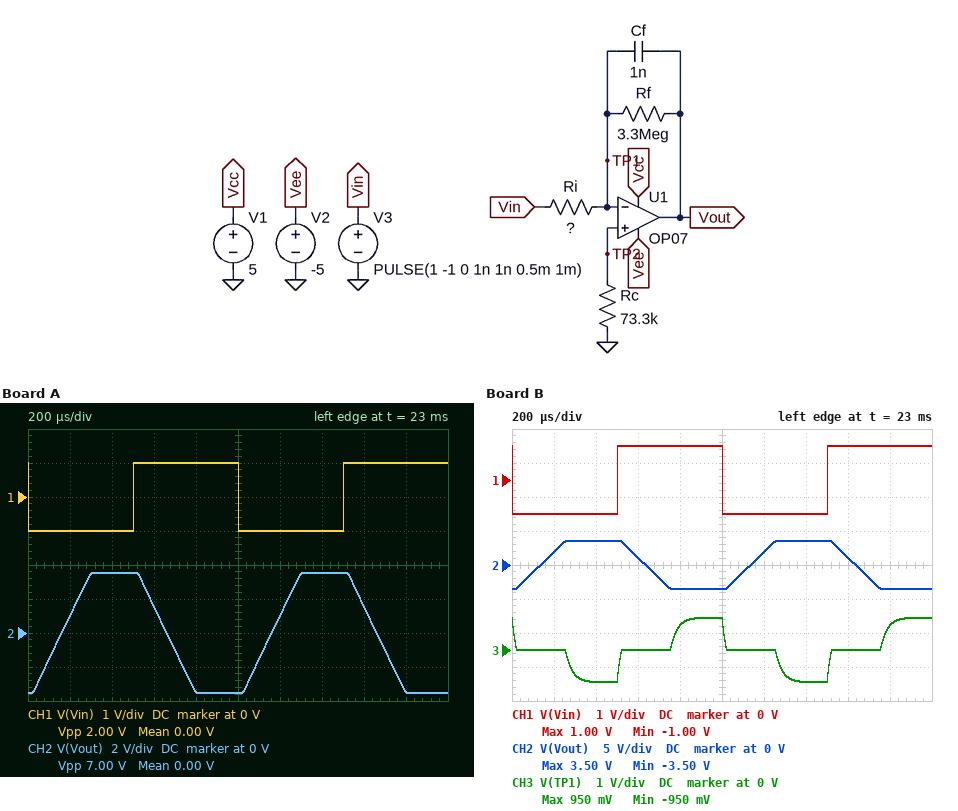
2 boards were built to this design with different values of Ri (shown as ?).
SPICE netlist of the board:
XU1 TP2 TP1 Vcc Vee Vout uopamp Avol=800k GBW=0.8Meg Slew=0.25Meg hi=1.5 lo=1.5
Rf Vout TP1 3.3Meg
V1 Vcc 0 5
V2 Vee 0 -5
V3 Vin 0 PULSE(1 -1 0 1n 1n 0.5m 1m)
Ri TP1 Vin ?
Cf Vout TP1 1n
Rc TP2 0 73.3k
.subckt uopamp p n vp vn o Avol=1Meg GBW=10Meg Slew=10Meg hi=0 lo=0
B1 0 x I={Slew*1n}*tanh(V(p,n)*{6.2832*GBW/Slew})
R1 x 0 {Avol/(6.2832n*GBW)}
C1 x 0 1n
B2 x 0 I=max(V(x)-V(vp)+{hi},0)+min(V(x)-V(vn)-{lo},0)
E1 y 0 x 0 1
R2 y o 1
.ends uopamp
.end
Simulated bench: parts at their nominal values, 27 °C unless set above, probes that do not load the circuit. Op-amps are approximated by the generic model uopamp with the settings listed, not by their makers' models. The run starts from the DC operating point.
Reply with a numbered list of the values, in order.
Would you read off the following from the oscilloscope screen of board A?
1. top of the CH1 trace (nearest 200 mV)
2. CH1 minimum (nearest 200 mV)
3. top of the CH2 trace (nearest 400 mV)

1. 1.0 V
2. -1.0 V
3. 3.6 V
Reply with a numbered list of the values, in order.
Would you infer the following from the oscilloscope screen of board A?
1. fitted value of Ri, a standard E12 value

1. 39 kΩ
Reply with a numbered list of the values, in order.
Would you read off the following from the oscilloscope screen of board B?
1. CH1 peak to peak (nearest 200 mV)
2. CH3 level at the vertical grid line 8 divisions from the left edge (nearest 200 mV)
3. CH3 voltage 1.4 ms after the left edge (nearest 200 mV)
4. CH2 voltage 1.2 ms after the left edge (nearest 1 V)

1. 2.0 V
2. 0 V
3. -1.0 V
4. 2 V
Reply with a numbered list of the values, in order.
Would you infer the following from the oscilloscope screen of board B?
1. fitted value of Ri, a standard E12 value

1. 33 kΩ
